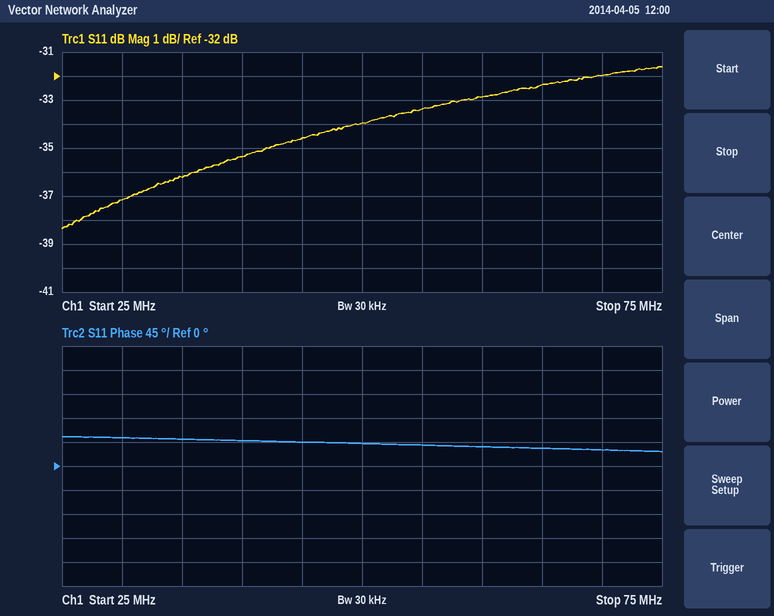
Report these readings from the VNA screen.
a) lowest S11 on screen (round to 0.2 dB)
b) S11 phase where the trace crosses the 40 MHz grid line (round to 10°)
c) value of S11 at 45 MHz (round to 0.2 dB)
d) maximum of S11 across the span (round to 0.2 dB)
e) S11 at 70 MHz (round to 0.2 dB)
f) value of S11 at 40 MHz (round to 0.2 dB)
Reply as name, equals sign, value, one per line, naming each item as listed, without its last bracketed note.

lowest S11 on screen = -38.4 dB
S11 phase where the trace crosses the 40 MHz grid line = 50°
value of S11 at 45 MHz = -34.6 dB
maximum of S11 across the span = -31.6 dB
S11 at 70 MHz = -32.0 dB
value of S11 at 40 MHz = -35.4 dB
